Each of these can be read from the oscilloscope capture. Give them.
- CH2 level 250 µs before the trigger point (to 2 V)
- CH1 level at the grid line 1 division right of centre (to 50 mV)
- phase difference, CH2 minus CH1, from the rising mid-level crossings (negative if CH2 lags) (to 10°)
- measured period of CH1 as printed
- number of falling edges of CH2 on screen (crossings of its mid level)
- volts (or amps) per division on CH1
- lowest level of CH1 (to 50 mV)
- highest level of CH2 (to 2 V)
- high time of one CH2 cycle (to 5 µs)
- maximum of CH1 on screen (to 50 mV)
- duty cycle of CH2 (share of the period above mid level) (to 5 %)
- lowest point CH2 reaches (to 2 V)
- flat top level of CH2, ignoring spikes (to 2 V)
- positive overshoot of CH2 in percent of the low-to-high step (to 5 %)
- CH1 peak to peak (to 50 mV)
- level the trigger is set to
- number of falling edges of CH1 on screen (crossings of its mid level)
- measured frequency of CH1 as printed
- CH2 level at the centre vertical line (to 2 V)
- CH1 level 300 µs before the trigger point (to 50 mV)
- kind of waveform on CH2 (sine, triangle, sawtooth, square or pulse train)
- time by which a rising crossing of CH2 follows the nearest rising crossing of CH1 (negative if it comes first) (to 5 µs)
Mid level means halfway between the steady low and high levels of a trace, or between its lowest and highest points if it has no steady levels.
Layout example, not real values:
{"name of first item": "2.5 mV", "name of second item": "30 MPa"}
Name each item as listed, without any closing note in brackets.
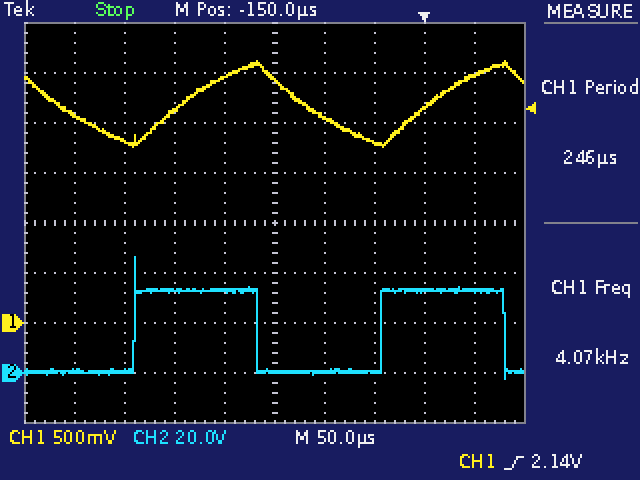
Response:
{"CH2 level 250 µs before the trigger point": "34 V", "CH1 level at the grid line 1 division right of centre": "2.05 V", "phase difference, CH2 minus CH1, from the rising mid-level crossings (negative if CH2 lags)": "+70°", "measured period of CH1 as printed": "246 µs", "number of falling edges of CH2 on screen": "2", "volts (or amps) per division on CH1": "500 mV", "lowest level of CH1": "1.75 V", "highest level of CH2": "46 V", "high time of one CH2 cycle": "125 µs", "maximum of CH1 on screen": "2.60 V", "duty cycle of CH2 (share of the period above mid level)": "50 %", "lowest point CH2 reaches": "-2 V", "flat top level of CH2, ignoring spikes": "34 V", "positive overshoot of CH2 in percent of the low-to-high step": "40 %", "CH1 peak to peak": "850 mV", "level the trigger is set to": "2.14 V", "number of falling edges of CH1 on screen": "2", "measured frequency of CH1 as printed": "4.07 kHz", "CH2 level at the centre vertical line": "0 V", "CH1 level 300 µs before the trigger point": "1.80 V", "kind of waveform on CH2": "square", "time by which a rising crossing of CH2 follows the nearest rising crossing of CH1 (negative if it comes first)": "-50 µs"}
